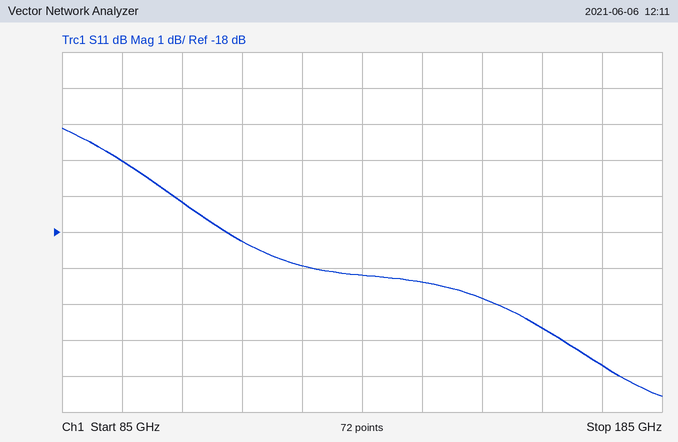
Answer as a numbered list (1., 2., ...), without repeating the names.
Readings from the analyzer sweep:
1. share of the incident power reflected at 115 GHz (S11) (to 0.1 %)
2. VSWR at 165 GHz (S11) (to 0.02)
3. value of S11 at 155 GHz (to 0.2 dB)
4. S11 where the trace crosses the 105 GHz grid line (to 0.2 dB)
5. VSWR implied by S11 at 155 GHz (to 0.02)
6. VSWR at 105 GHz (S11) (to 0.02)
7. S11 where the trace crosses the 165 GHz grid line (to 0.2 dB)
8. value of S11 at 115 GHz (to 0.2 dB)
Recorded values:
1. 1.5 %
2. 1.20
3. -19.8 dB
4. -17.2 dB
5. 1.22
6. 1.32
7. -20.6 dB
8. -18.2 dB
